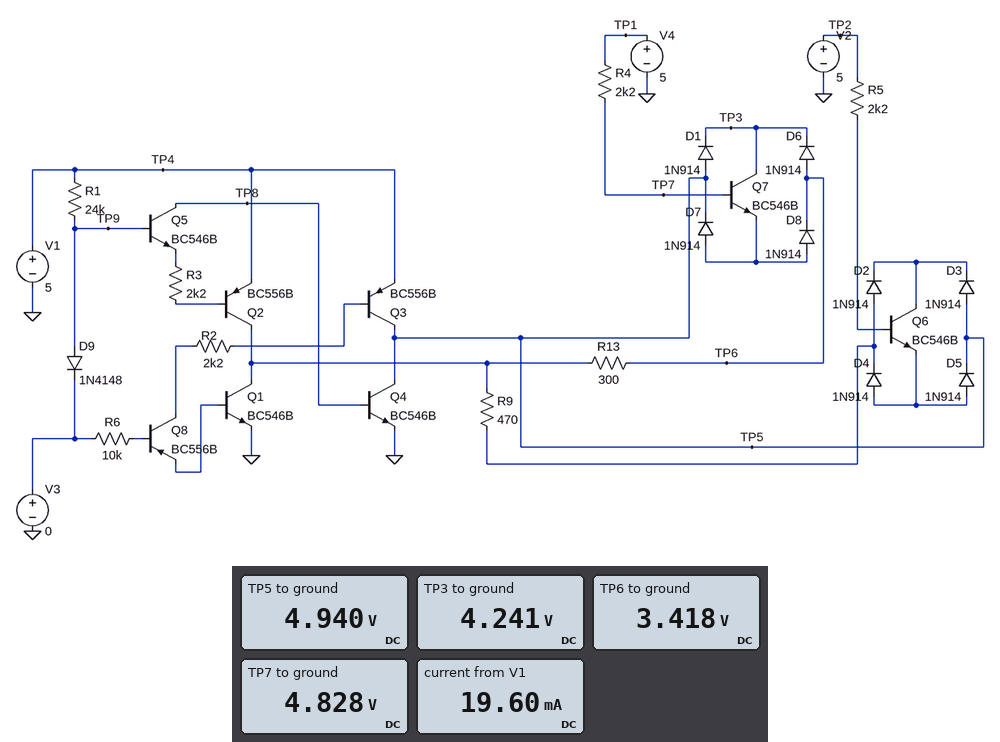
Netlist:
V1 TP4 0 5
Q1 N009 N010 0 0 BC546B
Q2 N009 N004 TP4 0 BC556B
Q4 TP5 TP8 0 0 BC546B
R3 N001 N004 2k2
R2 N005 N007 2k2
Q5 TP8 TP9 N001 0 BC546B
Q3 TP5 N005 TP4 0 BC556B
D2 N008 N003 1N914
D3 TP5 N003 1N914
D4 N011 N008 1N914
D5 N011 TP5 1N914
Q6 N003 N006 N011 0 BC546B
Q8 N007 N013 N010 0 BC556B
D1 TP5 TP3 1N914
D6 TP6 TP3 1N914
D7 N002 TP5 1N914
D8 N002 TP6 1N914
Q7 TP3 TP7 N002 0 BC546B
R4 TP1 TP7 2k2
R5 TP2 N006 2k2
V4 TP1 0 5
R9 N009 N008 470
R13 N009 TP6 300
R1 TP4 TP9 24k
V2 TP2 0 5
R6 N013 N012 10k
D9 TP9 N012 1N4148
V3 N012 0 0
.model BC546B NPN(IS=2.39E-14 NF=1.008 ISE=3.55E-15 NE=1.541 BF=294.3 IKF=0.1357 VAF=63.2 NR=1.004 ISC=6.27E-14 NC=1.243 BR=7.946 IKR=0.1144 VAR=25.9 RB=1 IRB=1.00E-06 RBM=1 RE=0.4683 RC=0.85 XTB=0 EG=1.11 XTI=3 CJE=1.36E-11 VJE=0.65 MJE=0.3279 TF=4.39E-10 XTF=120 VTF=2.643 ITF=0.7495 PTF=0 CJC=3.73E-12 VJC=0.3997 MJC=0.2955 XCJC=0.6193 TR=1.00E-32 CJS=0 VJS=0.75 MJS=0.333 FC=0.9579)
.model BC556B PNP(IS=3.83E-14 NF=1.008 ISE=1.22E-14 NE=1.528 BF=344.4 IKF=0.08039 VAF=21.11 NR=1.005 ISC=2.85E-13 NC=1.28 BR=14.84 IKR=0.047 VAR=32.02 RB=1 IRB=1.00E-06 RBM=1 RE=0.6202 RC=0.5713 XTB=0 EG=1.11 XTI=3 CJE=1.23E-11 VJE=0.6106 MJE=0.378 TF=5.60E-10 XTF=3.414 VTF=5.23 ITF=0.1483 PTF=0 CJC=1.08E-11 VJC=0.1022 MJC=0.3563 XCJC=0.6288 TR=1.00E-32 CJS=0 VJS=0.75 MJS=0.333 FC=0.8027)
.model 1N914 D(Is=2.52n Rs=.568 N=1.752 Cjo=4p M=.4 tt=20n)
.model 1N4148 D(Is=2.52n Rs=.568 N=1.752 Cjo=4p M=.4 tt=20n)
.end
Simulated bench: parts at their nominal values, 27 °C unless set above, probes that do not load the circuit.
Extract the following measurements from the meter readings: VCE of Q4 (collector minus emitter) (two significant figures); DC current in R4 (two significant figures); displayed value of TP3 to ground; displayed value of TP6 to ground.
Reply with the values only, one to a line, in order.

4.9 V
78 µA
4.241 V
3.418 V
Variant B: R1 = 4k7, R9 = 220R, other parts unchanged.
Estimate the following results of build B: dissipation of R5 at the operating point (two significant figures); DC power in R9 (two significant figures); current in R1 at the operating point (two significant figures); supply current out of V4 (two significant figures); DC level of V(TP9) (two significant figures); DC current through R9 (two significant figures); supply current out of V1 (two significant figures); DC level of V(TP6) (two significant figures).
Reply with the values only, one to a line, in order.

20 µW
49 mW
940 µA
84 µA
580 mV
15 mA
28 mA
3.4 V
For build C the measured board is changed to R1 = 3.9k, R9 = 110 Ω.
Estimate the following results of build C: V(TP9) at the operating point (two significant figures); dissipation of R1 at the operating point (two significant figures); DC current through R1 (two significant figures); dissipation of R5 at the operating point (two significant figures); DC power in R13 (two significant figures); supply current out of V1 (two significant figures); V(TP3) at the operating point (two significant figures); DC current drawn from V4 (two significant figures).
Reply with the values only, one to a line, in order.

590 mV
5.0 mW
1.1 mA
42 µW
36 mW
41 mA
4.2 V
94 µA
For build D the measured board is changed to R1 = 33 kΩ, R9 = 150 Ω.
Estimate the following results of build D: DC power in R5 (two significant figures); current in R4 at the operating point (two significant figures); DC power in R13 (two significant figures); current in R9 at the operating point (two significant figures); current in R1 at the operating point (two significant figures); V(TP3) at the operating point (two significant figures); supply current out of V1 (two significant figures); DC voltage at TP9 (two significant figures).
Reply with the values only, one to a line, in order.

29 µW
89 µA
36 mW
21 mA
140 µA
4.2 V
33 mA
490 mV
